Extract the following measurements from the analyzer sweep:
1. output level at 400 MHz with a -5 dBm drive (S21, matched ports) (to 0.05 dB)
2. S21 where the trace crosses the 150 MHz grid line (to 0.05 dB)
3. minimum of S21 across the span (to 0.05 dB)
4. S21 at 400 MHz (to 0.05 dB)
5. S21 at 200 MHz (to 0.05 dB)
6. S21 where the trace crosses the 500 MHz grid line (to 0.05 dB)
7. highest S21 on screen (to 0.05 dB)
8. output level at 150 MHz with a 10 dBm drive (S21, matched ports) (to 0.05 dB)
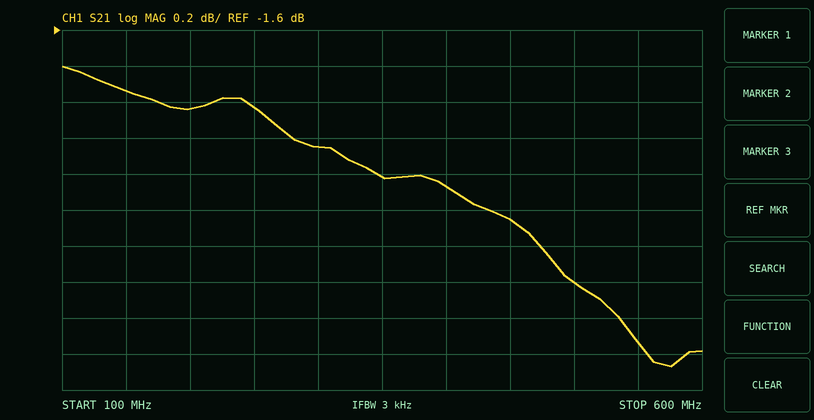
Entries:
-7.45 dBm
-1.95 dB
-3.45 dB
-2.45 dB
-2.05 dB
-3.00 dB
-1.80 dB
8.05 dBm
